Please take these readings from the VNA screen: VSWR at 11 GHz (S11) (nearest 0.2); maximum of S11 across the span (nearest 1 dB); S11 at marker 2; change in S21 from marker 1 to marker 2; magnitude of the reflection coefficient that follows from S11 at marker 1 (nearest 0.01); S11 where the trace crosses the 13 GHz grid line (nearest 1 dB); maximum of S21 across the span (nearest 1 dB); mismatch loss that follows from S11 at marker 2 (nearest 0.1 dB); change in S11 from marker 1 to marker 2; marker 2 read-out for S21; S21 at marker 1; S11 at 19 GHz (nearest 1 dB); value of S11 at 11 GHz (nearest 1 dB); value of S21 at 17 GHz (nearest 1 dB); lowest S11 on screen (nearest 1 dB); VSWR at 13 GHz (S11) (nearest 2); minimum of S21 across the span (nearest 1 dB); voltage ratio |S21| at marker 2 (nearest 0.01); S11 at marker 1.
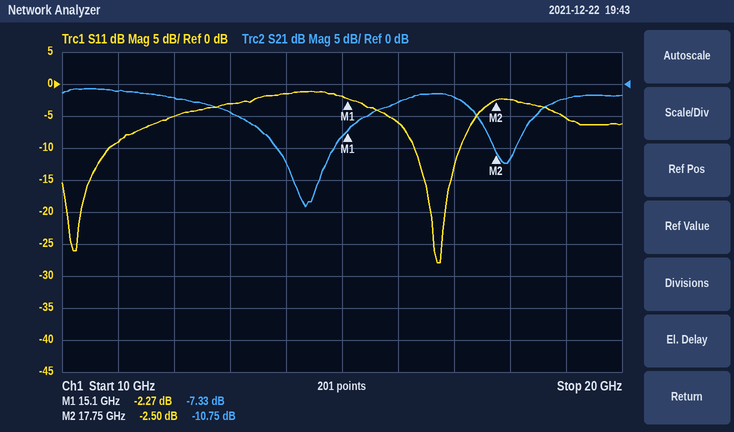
2.0
-1 dB
-2.50 dB
-3.42 dB
0.77
-3 dB
-1 dB
3.6 dB
-0.23 dB
-10.75 dB
-7.33 dB
-5 dB
-9 dB
-2 dB
-28 dB
6
-19 dB
0.29
-2.27 dB
